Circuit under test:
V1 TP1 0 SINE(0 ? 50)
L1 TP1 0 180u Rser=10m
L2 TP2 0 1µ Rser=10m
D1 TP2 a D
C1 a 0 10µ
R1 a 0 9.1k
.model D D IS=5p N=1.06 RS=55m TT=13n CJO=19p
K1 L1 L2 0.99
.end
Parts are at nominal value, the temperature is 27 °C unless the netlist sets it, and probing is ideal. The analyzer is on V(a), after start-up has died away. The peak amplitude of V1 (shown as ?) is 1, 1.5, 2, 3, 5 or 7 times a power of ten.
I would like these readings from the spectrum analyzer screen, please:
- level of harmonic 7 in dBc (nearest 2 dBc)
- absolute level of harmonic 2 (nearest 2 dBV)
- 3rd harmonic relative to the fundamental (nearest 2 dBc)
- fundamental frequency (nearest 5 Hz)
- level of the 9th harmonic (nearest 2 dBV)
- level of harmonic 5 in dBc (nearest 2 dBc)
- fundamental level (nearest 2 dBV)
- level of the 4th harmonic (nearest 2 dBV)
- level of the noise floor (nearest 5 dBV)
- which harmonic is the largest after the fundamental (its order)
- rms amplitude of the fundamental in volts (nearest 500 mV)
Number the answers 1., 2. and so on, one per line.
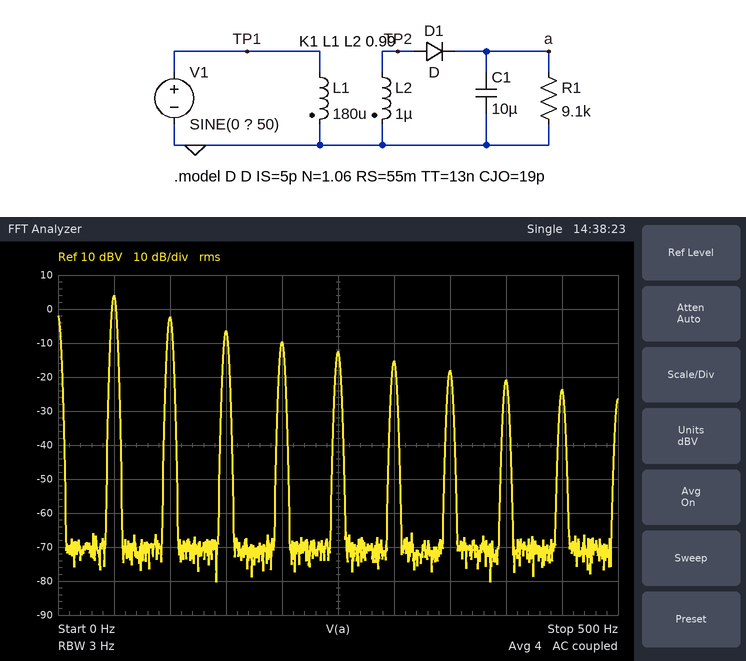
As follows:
1. -22 dBc
2. -2 dBV
3. -10 dBc
4. 50 Hz
5. -24 dBV
6. -16 dBc
7. 4 dBV
8. -10 dBV
9. -70 dBV
10. 2
11. 1.5 V
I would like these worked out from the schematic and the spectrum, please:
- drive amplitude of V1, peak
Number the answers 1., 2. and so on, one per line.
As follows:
1. 500 V
